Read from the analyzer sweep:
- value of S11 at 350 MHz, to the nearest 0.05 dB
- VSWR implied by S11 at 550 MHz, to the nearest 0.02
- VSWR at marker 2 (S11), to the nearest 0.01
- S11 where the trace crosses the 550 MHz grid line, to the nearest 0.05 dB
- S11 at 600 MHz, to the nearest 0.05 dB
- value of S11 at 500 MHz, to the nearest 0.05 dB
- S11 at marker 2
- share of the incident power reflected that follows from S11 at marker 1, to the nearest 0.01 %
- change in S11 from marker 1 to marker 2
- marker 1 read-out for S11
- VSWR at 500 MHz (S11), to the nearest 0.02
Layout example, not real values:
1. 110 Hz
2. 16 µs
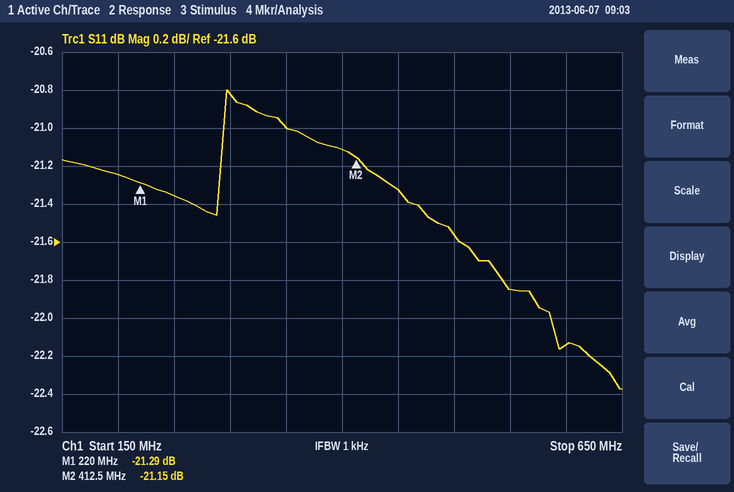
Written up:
1. -21.00 dB
2. 1.18
3. 1.19
4. -21.85 dB
5. -22.15 dB
6. -21.55 dB
7. -21.15 dB
8. 0.74 %
9. 0.14 dB
10. -21.29 dB
11. 1.18
